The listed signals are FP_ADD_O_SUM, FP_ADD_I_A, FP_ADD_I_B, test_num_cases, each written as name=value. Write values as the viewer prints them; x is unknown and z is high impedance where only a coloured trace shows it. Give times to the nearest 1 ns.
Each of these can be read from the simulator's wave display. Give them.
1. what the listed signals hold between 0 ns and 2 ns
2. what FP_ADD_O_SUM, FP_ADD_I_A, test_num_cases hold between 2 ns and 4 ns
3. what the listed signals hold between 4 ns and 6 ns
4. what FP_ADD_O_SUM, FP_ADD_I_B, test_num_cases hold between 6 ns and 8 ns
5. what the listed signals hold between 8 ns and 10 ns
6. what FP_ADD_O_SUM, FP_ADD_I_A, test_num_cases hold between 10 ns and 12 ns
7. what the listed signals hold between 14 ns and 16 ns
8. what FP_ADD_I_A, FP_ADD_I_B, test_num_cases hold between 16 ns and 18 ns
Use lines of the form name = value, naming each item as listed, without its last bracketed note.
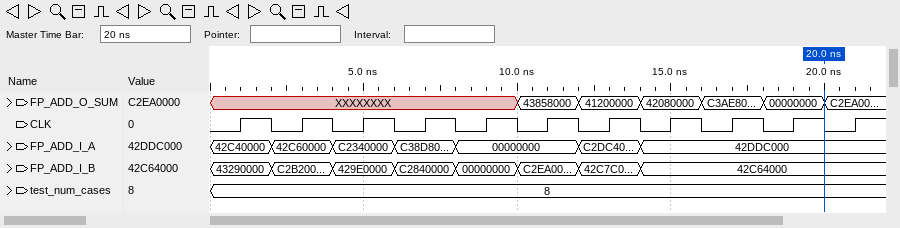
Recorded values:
what the listed signals hold between 0 ns and 2 ns = FP_ADD_O_SUM=XXXXXXXX, FP_ADD_I_A=42C40000, FP_ADD_I_B=43290000, test_num_cases=8
what FP_ADD_O_SUM, FP_ADD_I_A, test_num_cases hold between 2 ns and 4 ns = FP_ADD_O_SUM=XXXXXXXX, FP_ADD_I_A=42C60000, test_num_cases=8
what the listed signals hold between 4 ns and 6 ns = FP_ADD_O_SUM=XXXXXXXX, FP_ADD_I_A=C2340000, FP_ADD_I_B=429E0000, test_num_cases=8
what FP_ADD_O_SUM, FP_ADD_I_B, test_num_cases hold between 6 ns and 8 ns = FP_ADD_O_SUM=XXXXXXXX, FP_ADD_I_B=C2840000, test_num_cases=8
what the listed signals hold between 8 ns and 10 ns = FP_ADD_O_SUM=XXXXXXXX, FP_ADD_I_A=00000000, FP_ADD_I_B=00000000, test_num_cases=8
what FP_ADD_O_SUM, FP_ADD_I_A, test_num_cases hold between 10 ns and 12 ns = FP_ADD_O_SUM=43858000, FP_ADD_I_A=00000000, test_num_cases=8
what the listed signals hold between 14 ns and 16 ns = FP_ADD_O_SUM=42080000, FP_ADD_I_A=42DDC000, FP_ADD_I_B=42C64000, test_num_cases=8
what FP_ADD_I_A, FP_ADD_I_B, test_num_cases hold between 16 ns and 18 ns = FP_ADD_I_A=42DDC000, FP_ADD_I_B=42C64000, test_num_cases=8
